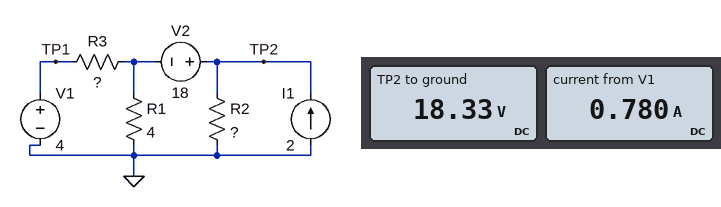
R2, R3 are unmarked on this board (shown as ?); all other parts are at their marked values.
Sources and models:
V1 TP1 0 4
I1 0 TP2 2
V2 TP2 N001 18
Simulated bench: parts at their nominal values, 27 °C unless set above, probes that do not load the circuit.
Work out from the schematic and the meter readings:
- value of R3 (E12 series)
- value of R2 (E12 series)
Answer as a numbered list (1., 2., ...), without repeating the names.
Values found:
1. 4.7 Ω
2. 6.8 Ω
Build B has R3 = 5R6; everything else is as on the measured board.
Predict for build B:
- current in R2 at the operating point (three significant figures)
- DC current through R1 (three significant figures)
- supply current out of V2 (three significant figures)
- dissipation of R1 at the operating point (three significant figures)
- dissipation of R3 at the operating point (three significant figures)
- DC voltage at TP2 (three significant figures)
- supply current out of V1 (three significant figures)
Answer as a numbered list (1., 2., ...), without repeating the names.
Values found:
1. 2.66 A
2. 29.2 mA
3. 664 mA
4. 3.41 mW
5. 2.69 W
6. 18.1 V
7. 693 mA
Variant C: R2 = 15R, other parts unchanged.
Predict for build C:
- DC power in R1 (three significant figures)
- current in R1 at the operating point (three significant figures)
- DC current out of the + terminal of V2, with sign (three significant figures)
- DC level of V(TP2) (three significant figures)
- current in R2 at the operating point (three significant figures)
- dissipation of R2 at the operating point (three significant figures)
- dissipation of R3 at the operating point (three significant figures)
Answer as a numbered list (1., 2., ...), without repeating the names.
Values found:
1. 2.43 W
2. 780 mA
3. -592 mA
4. 21.1 V
5. 1.41 A
6. 29.7 W
7. 165 mW
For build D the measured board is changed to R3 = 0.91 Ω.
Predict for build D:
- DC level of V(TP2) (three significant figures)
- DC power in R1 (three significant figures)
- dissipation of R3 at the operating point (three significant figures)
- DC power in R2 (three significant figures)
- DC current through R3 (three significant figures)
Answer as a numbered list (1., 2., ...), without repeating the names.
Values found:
1. 20.5 V
2. 1.57 W
3. 2.45 W
4. 61.8 W
5. 1.64 A
